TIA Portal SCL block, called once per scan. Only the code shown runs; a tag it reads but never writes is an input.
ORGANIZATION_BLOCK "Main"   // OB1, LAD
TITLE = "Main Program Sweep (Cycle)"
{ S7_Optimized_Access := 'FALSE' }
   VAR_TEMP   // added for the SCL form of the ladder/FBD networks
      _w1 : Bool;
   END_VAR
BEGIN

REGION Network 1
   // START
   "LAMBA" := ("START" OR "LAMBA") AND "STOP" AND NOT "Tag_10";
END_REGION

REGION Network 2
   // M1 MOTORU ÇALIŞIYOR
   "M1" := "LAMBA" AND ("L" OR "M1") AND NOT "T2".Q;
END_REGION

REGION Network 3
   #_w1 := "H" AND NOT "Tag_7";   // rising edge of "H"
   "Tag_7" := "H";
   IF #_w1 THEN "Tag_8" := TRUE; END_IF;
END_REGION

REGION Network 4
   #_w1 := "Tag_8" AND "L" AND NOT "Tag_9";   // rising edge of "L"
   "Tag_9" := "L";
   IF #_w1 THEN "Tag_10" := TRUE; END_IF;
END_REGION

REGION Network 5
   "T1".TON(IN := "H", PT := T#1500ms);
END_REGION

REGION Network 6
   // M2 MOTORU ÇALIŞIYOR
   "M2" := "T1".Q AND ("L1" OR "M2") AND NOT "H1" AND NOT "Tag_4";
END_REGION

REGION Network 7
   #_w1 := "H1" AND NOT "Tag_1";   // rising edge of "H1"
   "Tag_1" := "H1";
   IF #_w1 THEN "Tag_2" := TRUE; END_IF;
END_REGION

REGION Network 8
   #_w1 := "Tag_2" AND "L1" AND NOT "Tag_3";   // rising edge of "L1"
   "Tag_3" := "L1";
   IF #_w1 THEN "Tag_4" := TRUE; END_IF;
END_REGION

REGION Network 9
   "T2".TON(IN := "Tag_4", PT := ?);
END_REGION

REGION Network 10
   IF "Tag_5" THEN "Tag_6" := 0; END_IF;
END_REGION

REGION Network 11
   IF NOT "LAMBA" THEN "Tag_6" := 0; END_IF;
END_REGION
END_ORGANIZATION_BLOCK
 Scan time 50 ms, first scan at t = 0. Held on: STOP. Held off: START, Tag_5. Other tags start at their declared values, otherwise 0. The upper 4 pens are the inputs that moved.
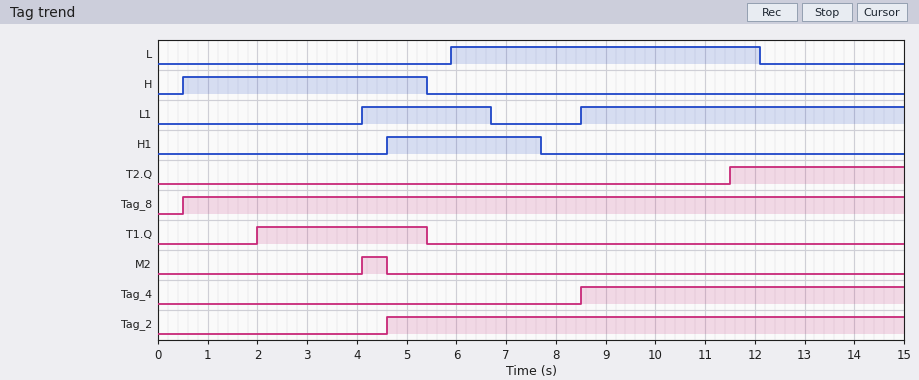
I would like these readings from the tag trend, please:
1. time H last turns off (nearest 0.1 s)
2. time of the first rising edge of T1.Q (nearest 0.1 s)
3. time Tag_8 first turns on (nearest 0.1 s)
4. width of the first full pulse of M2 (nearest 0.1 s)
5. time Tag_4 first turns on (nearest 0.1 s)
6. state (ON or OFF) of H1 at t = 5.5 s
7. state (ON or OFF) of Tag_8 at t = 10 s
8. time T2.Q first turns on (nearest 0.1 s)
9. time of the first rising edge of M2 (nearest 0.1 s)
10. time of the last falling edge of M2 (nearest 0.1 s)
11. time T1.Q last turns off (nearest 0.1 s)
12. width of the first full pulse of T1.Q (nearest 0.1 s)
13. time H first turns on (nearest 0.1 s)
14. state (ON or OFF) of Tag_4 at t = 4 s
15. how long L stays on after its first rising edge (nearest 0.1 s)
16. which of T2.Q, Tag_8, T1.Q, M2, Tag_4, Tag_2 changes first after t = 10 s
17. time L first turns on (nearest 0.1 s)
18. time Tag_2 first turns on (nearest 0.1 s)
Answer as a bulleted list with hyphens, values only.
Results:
- 5.4 s
- 2.0 s
- 0.5 s
- 0.5 s
- 8.5 s
- ON
- ON
- 11.5 s
- 4.1 s
- 4.6 s
- 5.4 s
- 3.4 s
- 0.5 s
- OFF
- 6.2 s
- T2.Q
- 5.9 s
- 4.6 s
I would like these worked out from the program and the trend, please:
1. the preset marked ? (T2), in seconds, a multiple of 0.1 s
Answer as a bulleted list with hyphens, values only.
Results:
- 3.0 s
